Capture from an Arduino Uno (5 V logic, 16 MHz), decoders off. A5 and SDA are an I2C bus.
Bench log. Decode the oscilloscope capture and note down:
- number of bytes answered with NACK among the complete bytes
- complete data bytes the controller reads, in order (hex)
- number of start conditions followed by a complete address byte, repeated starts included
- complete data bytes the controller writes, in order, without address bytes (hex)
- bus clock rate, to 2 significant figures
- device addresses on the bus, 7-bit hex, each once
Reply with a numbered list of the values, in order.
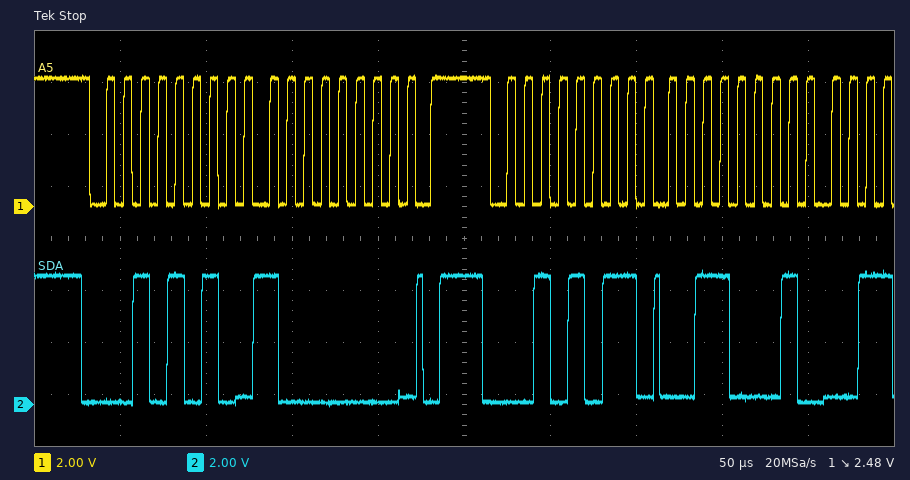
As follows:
1. 0
2. 31
3. 2
4. 80
5. 100 kHz
6. 0x15
